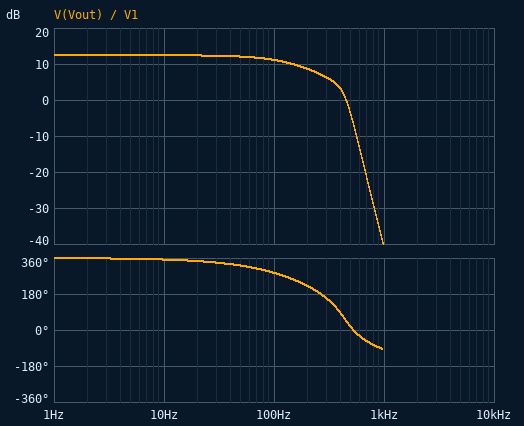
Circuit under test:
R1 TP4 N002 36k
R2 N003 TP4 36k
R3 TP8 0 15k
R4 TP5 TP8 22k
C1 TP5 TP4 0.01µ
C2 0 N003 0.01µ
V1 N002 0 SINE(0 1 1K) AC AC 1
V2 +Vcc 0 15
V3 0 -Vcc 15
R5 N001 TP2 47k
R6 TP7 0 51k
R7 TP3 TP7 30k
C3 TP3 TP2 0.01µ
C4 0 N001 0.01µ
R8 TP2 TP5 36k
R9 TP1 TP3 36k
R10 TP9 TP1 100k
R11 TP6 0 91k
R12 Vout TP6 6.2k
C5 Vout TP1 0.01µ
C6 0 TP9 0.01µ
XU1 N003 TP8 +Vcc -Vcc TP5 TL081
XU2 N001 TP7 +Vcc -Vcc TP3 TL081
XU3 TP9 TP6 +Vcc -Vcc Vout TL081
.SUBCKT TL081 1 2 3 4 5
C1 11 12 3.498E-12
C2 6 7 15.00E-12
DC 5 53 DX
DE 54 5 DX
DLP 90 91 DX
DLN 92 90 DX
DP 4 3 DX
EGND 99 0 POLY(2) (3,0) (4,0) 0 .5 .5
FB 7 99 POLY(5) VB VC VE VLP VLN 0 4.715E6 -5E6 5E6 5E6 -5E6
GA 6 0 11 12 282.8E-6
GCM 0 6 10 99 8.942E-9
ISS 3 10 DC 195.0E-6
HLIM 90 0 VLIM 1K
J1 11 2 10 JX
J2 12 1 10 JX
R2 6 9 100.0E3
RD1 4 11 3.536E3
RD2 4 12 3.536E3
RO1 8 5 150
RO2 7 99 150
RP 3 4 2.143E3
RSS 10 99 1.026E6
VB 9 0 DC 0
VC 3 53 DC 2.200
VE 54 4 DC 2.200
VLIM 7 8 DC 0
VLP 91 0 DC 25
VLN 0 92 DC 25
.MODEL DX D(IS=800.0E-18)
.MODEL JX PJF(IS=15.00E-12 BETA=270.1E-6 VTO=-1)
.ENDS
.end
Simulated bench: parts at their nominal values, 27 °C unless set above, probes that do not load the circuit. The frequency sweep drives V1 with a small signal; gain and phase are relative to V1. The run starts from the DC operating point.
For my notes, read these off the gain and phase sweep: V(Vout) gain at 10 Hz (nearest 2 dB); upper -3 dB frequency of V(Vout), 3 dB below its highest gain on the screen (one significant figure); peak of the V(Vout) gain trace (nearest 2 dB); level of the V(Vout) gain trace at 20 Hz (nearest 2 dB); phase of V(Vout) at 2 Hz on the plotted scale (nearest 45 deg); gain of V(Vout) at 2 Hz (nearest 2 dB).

12 dB
200 Hz
12 dB
12 dB
360 deg
12 dB
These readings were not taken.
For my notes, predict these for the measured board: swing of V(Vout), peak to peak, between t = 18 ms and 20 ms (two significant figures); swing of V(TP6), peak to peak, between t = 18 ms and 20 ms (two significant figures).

18 mV
17 mV
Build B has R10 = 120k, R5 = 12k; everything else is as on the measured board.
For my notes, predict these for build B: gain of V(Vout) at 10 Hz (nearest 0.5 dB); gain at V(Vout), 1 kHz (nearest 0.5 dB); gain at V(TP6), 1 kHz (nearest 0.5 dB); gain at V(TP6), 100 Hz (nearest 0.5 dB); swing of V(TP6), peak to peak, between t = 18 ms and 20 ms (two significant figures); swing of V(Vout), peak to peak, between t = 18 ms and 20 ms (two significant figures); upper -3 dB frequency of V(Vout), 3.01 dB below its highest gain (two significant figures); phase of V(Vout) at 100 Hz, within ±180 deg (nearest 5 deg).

12.5 dB
-31.0 dB
-31.5 dB
10.0 dB
53 mV
57 mV
150 Hz
-65 deg
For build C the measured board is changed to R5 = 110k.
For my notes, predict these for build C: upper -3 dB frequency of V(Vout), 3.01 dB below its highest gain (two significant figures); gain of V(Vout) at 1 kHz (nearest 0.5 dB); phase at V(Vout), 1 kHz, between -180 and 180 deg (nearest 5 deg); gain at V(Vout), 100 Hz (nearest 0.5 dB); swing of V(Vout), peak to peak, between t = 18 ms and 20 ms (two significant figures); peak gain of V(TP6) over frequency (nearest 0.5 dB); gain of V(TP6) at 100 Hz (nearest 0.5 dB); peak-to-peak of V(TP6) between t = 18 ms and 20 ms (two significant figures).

110 Hz
-48.5 dB
-105 deg
10.0 dB
7.5 mV
12.0 dB
9.5 dB
7.0 mV
